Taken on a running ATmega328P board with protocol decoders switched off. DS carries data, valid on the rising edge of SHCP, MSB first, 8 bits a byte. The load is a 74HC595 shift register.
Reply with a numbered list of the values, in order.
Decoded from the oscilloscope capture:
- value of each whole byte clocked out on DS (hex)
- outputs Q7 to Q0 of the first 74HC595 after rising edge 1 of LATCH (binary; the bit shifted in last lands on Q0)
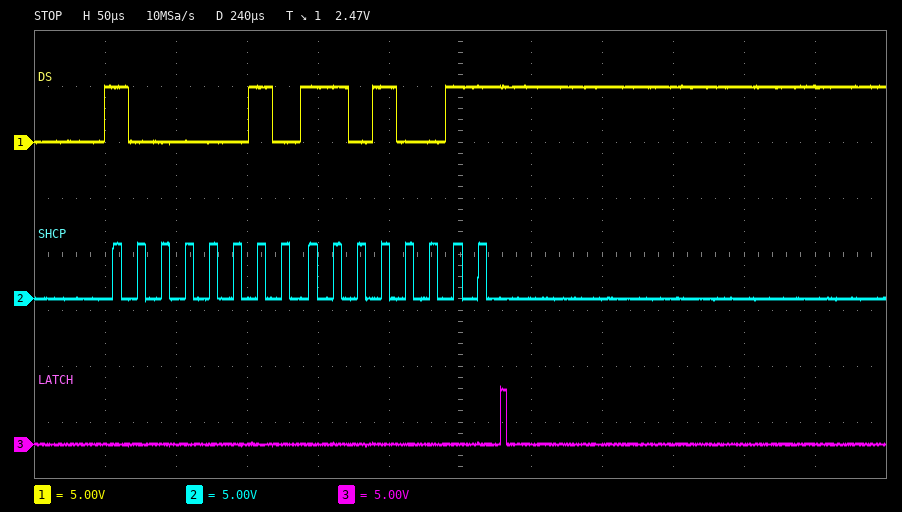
1. 82 D3
2. 11010011
